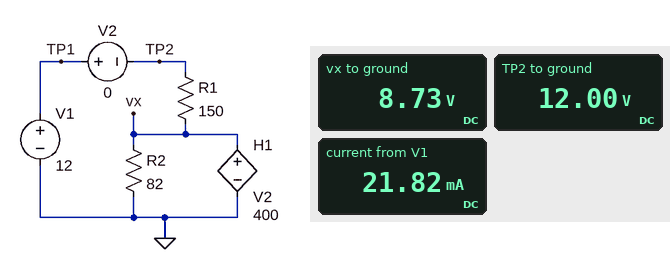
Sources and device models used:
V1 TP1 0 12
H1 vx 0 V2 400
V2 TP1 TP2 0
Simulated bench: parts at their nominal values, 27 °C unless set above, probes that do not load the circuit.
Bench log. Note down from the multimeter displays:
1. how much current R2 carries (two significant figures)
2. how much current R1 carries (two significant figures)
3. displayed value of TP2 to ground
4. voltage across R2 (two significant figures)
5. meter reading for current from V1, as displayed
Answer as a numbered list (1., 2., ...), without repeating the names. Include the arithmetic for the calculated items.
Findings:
1. (8.73 V) / 82 Ω = 110 mA
2. (12 V - 8.73 V) / 150 Ω = 22 mA
3. 12.00 V
4. 8.73 V = 8.7 V
5. 21.82 mA
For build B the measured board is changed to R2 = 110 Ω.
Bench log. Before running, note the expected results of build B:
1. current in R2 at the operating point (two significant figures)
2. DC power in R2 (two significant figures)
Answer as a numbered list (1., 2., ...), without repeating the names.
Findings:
1. 79 mA
2. 690 mW
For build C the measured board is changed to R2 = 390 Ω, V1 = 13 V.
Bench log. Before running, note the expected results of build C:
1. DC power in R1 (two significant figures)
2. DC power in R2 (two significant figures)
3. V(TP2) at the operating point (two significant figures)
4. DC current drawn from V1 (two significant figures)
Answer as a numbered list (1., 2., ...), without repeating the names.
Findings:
1. 84 mW
2. 230 mW
3. 13 V
4. 24 mA
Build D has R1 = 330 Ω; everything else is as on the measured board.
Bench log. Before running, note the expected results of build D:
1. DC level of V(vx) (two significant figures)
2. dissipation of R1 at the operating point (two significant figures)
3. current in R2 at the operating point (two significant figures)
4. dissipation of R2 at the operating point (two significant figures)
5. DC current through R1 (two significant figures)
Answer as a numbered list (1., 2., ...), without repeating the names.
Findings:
1. 6.6 V
2. 89 mW
3. 80 mA
4. 530 mW
5. 16 mA
